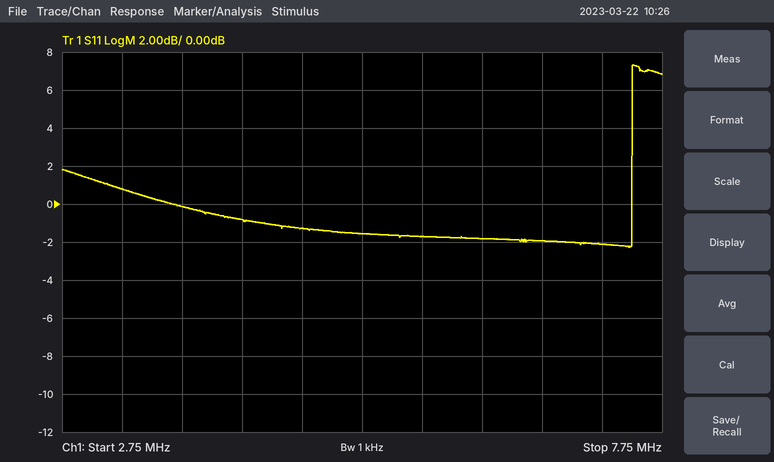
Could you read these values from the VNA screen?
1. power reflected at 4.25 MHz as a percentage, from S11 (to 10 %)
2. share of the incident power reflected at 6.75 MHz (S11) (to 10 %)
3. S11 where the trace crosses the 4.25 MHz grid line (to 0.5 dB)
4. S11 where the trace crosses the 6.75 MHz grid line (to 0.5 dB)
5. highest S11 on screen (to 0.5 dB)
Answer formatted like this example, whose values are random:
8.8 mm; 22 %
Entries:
80 %; 60 %; -1.0 dB; -2.0 dB; 7.5 dB
